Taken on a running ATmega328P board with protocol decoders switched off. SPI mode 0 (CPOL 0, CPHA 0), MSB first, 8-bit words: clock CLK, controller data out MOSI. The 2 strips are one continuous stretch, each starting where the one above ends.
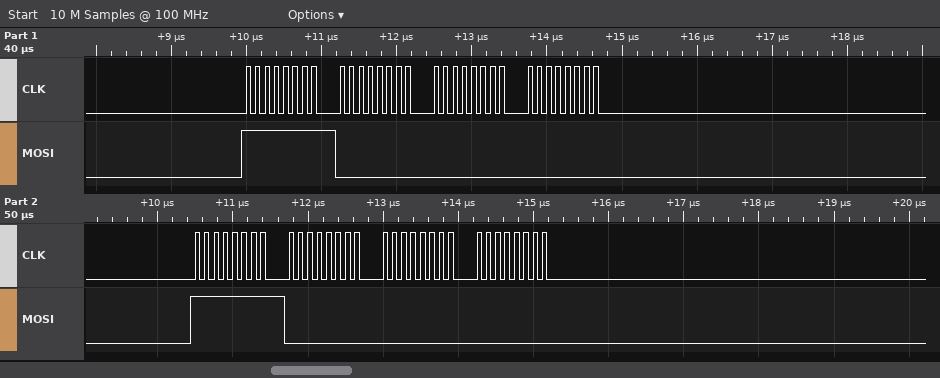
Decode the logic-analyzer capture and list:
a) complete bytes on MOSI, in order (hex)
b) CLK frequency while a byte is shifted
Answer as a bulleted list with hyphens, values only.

- FF 00 00 00 FF 00 00 00
- 8 MHz
